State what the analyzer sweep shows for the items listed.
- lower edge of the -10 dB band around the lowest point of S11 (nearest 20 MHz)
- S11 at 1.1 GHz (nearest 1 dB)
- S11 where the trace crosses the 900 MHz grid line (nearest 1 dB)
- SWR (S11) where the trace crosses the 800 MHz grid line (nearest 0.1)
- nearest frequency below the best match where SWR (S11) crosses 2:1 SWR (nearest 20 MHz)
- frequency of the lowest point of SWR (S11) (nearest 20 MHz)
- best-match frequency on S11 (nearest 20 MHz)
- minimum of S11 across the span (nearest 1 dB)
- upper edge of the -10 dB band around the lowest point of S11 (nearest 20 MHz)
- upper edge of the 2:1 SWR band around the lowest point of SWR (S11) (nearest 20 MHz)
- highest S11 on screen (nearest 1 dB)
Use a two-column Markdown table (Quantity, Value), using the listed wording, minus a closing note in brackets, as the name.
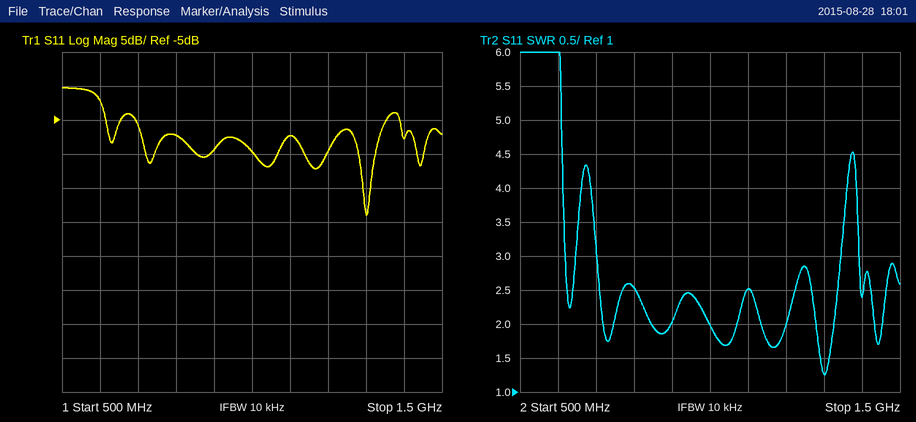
| Quantity | Value |
|---|---|
| lower edge of the -10 dB band around the lowest point of S11 | 1.28 GHz |
| S11 at 1.1 GHz | -7 dB |
| S11 where the trace crosses the 900 MHz grid line | -9 dB |
| SWR (S11) where the trace crosses the 800 MHz grid line | 2.5 |
| nearest frequency below the best match where SWR (S11) crosses 2:1 SWR | 1.28 GHz |
| frequency of the lowest point of SWR (S11) | 1.30 GHz |
| best-match frequency on S11 | 1.30 GHz |
| minimum of S11 across the span | -19 dB |
| upper edge of the -10 dB band around the lowest point of S11 | 1.32 GHz |
| upper edge of the 2:1 SWR band around the lowest point of SWR (S11) | 1.32 GHz |
| highest S11 on screen | 0 dB |
